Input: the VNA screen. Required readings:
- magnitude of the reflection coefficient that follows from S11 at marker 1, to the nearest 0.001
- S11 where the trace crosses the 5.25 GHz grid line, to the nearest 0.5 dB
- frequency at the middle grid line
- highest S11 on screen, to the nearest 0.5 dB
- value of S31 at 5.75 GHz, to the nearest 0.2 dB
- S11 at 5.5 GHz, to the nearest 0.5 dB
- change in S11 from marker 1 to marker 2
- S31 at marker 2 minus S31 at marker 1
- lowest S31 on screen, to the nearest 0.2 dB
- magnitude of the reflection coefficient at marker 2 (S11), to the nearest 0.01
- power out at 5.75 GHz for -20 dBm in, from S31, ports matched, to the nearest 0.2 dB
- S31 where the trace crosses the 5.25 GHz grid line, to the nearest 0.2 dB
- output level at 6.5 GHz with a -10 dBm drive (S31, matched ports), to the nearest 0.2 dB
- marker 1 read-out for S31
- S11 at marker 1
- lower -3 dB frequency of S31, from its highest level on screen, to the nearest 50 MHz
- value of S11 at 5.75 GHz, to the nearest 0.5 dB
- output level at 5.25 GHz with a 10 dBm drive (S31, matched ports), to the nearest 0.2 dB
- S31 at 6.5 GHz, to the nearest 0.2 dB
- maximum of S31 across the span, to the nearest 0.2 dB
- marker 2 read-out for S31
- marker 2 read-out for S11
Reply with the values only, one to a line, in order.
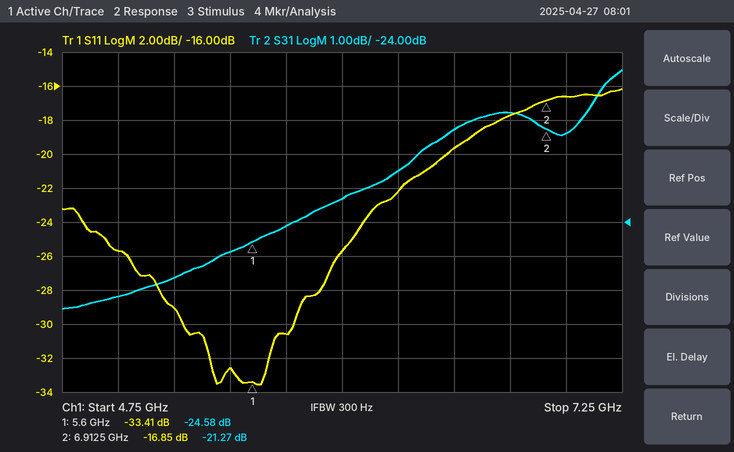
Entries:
0.021
-29.0 dB
6 GHz
-16.0 dB
-24.2 dB
-32.5 dB
16.56 dB
3.31 dB
-26.6 dB
0.14
-44.2 dBm
-25.6 dB
-31.2 dBm
-24.58 dB
-33.41 dB
6.25 GHz
-30.5 dB
-15.6 dBm
-21.2 dB
-19.6 dB
-21.27 dB
-16.85 dB
